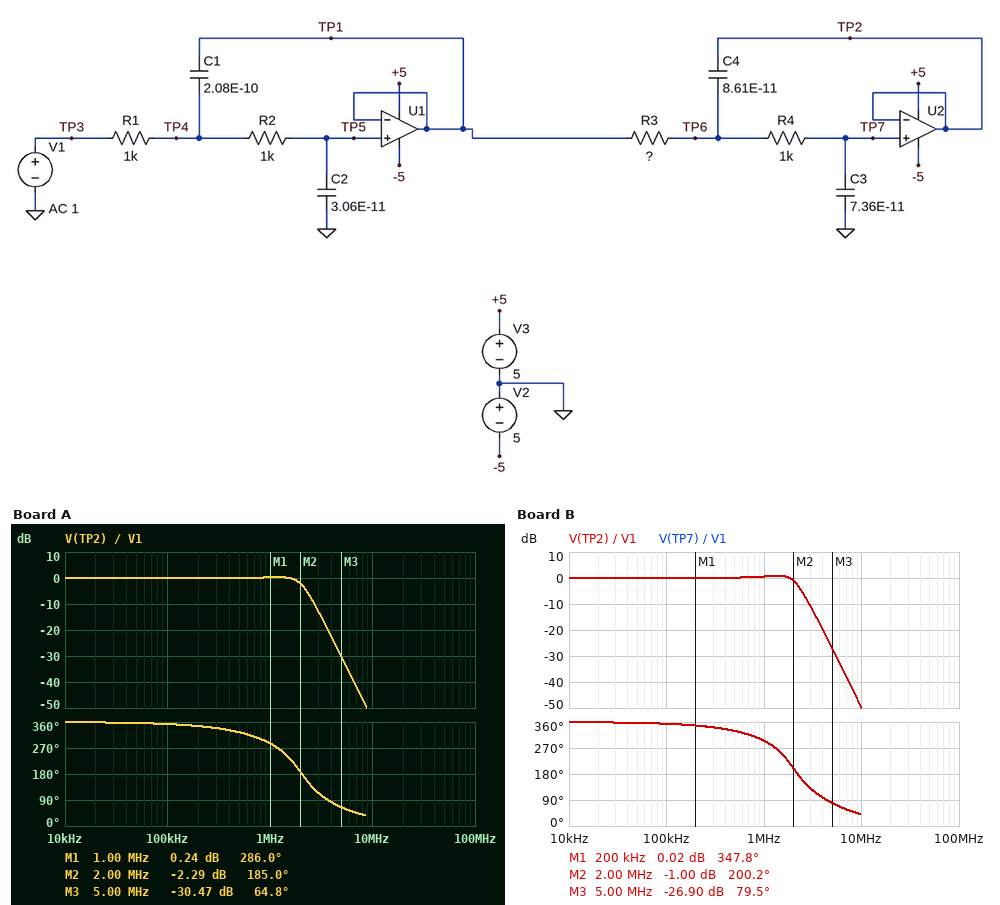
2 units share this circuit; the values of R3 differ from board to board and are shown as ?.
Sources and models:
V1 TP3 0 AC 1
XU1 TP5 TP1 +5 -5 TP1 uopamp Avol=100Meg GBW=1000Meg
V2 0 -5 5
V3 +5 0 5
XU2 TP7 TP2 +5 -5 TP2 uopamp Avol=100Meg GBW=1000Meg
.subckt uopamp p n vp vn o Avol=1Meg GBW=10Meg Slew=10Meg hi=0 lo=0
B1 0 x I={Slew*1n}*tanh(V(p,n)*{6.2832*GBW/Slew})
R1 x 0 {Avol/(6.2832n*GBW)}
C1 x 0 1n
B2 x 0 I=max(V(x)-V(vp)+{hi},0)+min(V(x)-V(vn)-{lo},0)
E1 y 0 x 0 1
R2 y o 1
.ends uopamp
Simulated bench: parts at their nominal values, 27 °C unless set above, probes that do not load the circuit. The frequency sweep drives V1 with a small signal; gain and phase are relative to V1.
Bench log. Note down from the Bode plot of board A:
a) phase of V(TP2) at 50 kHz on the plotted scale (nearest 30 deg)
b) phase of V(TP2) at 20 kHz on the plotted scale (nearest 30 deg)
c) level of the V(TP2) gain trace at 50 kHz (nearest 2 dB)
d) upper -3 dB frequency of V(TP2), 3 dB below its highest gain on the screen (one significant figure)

360 deg
360 deg
0 dB
2 MHz
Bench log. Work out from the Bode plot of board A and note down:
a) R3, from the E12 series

820 Ω
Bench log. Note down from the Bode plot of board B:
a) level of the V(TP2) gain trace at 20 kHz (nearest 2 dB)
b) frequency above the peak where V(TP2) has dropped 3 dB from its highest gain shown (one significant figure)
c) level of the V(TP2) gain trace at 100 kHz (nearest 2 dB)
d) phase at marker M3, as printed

0 dB
2 MHz
0 dB
79.5 deg
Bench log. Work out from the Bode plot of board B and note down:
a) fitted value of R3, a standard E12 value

470 Ω
